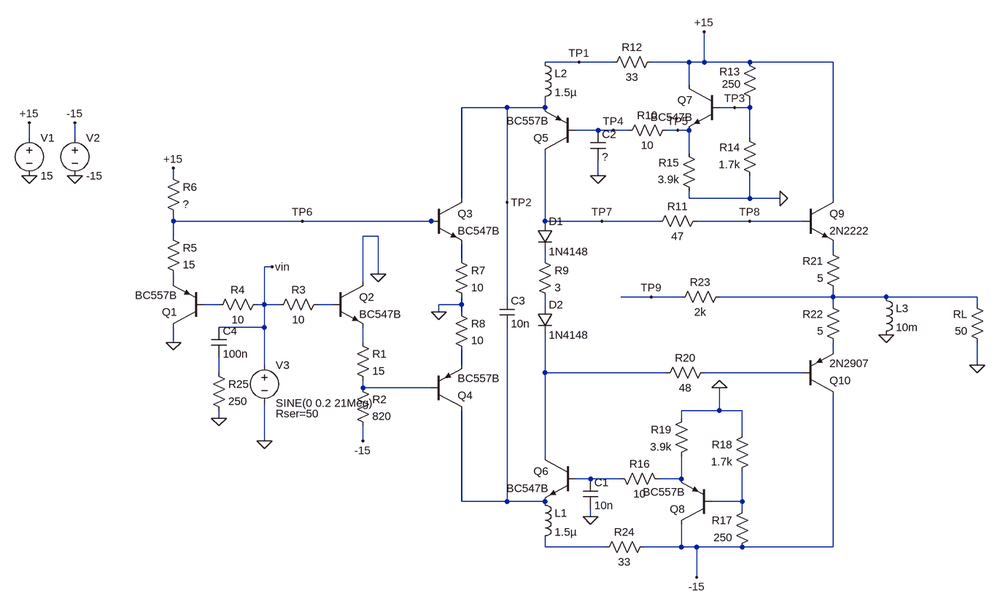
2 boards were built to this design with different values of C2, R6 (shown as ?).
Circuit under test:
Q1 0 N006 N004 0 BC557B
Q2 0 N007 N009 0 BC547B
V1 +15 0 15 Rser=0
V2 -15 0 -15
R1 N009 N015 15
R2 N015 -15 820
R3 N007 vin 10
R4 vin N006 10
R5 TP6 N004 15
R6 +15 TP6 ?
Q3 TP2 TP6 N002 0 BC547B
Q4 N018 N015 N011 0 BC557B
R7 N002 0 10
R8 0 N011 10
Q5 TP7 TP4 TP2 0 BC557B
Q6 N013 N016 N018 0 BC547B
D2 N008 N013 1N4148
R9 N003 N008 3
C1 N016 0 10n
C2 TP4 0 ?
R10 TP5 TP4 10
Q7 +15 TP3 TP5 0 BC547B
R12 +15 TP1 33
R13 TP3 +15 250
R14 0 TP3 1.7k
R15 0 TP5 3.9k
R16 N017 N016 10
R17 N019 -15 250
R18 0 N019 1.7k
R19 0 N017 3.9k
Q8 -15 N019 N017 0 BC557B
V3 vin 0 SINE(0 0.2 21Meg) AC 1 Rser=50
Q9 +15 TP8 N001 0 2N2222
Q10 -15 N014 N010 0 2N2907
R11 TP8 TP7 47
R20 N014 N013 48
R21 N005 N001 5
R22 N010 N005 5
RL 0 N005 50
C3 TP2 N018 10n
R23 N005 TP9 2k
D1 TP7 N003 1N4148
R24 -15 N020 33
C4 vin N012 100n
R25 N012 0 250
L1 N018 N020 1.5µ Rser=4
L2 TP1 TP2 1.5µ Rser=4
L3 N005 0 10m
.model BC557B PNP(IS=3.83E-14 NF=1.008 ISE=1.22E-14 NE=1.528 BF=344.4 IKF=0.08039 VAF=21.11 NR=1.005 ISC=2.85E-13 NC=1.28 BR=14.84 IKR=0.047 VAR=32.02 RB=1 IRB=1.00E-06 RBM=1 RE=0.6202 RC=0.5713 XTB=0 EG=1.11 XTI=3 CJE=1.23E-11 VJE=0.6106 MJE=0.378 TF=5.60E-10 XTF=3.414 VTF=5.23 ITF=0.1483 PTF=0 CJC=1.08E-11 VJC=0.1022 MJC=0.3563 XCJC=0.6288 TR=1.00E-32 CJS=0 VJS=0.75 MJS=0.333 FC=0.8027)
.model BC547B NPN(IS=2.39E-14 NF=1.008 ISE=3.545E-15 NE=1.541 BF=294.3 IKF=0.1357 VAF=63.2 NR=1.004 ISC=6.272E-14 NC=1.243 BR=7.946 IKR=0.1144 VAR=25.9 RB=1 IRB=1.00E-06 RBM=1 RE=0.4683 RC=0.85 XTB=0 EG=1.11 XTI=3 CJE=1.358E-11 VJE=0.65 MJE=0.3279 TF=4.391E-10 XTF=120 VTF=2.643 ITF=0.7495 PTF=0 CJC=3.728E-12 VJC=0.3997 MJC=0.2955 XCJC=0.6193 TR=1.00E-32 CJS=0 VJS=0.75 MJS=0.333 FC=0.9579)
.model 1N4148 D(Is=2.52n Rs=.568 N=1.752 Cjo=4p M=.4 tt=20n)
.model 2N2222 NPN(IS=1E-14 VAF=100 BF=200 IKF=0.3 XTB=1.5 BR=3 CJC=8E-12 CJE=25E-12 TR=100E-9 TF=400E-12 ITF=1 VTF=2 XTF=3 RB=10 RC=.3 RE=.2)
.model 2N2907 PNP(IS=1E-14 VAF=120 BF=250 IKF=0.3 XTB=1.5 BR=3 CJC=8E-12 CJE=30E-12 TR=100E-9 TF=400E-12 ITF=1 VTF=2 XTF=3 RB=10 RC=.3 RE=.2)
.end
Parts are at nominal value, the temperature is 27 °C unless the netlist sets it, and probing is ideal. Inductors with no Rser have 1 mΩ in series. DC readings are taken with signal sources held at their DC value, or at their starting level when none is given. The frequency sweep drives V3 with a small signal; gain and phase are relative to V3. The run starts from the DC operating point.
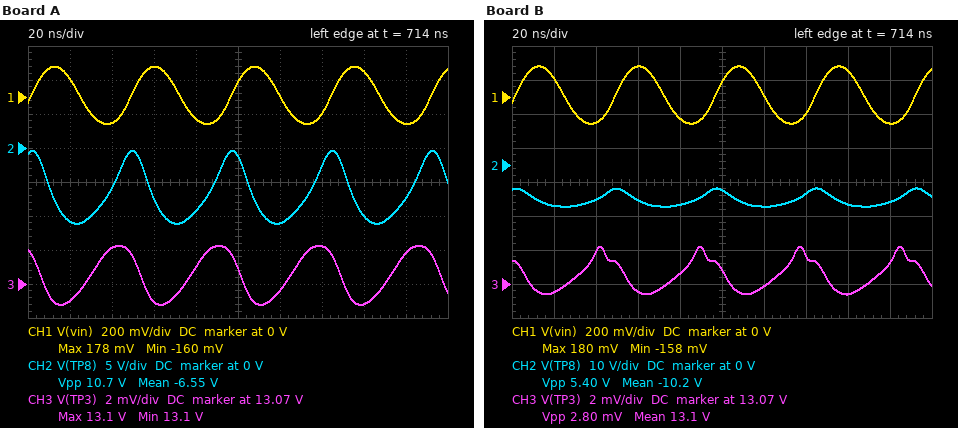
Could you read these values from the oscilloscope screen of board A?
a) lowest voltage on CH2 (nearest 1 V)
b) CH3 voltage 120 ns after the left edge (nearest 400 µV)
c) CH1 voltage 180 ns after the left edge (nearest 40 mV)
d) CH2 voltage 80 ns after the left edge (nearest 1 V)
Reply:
-11 V
13.0736 V
-160 mV
-9 V
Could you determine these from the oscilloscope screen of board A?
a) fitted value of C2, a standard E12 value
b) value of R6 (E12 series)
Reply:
4.7 nF
390 Ω
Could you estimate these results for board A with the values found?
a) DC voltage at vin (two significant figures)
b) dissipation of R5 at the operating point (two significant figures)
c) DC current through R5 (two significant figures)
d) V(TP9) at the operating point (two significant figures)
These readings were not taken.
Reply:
4.2 mV
18 mW
35 mA
-1.2 mV
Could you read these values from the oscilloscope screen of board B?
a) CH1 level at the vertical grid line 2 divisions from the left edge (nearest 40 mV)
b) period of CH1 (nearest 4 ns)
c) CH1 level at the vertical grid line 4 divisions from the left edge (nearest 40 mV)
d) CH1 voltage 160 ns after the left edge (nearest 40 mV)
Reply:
-160 mV
48 ns
-120 mV
160 mV
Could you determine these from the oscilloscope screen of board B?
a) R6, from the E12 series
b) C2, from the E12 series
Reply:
330 Ω
3.3 nF
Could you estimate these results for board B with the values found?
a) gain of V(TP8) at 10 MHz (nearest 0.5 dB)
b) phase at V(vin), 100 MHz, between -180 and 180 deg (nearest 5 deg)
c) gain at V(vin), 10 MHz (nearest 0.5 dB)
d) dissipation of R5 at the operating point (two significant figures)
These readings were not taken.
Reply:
29.5 dB
-55 deg
-1.5 dB
25 mW
